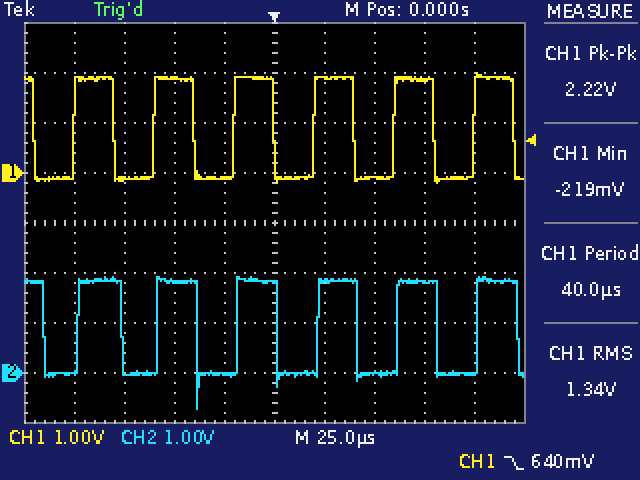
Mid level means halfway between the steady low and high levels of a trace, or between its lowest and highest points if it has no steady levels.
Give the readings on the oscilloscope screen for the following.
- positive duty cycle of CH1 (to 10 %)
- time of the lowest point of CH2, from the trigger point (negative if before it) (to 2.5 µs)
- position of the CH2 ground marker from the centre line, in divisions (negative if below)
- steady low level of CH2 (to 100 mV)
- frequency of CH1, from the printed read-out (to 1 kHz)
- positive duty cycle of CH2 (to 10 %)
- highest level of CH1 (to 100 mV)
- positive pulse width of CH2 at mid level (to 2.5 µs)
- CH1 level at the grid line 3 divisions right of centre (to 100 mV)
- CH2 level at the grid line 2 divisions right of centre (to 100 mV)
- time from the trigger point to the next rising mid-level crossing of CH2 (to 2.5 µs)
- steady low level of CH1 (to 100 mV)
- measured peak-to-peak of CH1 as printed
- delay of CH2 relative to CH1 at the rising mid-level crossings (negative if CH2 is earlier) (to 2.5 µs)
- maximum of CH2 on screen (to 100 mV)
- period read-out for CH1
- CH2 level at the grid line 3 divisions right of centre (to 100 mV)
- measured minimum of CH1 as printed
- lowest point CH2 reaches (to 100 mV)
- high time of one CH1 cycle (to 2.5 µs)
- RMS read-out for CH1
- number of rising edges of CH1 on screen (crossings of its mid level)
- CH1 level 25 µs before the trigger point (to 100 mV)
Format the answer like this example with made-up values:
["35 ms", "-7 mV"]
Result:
["50 %", "-37.5 µs", "-3.0 div", "0.0 V", "25 kHz", "50 %", "2.0 V", "20.0 µs", "1.9 V", "0.0 V", "22.5 µs", "-100 mV", "2.22 V", "+2.5 µs", "1.9 V", "40.0 µs", "1.8 V", "-219 mV", "-700 mV", "20.0 µs", "1.34 V", "6", "-100 mV"]
